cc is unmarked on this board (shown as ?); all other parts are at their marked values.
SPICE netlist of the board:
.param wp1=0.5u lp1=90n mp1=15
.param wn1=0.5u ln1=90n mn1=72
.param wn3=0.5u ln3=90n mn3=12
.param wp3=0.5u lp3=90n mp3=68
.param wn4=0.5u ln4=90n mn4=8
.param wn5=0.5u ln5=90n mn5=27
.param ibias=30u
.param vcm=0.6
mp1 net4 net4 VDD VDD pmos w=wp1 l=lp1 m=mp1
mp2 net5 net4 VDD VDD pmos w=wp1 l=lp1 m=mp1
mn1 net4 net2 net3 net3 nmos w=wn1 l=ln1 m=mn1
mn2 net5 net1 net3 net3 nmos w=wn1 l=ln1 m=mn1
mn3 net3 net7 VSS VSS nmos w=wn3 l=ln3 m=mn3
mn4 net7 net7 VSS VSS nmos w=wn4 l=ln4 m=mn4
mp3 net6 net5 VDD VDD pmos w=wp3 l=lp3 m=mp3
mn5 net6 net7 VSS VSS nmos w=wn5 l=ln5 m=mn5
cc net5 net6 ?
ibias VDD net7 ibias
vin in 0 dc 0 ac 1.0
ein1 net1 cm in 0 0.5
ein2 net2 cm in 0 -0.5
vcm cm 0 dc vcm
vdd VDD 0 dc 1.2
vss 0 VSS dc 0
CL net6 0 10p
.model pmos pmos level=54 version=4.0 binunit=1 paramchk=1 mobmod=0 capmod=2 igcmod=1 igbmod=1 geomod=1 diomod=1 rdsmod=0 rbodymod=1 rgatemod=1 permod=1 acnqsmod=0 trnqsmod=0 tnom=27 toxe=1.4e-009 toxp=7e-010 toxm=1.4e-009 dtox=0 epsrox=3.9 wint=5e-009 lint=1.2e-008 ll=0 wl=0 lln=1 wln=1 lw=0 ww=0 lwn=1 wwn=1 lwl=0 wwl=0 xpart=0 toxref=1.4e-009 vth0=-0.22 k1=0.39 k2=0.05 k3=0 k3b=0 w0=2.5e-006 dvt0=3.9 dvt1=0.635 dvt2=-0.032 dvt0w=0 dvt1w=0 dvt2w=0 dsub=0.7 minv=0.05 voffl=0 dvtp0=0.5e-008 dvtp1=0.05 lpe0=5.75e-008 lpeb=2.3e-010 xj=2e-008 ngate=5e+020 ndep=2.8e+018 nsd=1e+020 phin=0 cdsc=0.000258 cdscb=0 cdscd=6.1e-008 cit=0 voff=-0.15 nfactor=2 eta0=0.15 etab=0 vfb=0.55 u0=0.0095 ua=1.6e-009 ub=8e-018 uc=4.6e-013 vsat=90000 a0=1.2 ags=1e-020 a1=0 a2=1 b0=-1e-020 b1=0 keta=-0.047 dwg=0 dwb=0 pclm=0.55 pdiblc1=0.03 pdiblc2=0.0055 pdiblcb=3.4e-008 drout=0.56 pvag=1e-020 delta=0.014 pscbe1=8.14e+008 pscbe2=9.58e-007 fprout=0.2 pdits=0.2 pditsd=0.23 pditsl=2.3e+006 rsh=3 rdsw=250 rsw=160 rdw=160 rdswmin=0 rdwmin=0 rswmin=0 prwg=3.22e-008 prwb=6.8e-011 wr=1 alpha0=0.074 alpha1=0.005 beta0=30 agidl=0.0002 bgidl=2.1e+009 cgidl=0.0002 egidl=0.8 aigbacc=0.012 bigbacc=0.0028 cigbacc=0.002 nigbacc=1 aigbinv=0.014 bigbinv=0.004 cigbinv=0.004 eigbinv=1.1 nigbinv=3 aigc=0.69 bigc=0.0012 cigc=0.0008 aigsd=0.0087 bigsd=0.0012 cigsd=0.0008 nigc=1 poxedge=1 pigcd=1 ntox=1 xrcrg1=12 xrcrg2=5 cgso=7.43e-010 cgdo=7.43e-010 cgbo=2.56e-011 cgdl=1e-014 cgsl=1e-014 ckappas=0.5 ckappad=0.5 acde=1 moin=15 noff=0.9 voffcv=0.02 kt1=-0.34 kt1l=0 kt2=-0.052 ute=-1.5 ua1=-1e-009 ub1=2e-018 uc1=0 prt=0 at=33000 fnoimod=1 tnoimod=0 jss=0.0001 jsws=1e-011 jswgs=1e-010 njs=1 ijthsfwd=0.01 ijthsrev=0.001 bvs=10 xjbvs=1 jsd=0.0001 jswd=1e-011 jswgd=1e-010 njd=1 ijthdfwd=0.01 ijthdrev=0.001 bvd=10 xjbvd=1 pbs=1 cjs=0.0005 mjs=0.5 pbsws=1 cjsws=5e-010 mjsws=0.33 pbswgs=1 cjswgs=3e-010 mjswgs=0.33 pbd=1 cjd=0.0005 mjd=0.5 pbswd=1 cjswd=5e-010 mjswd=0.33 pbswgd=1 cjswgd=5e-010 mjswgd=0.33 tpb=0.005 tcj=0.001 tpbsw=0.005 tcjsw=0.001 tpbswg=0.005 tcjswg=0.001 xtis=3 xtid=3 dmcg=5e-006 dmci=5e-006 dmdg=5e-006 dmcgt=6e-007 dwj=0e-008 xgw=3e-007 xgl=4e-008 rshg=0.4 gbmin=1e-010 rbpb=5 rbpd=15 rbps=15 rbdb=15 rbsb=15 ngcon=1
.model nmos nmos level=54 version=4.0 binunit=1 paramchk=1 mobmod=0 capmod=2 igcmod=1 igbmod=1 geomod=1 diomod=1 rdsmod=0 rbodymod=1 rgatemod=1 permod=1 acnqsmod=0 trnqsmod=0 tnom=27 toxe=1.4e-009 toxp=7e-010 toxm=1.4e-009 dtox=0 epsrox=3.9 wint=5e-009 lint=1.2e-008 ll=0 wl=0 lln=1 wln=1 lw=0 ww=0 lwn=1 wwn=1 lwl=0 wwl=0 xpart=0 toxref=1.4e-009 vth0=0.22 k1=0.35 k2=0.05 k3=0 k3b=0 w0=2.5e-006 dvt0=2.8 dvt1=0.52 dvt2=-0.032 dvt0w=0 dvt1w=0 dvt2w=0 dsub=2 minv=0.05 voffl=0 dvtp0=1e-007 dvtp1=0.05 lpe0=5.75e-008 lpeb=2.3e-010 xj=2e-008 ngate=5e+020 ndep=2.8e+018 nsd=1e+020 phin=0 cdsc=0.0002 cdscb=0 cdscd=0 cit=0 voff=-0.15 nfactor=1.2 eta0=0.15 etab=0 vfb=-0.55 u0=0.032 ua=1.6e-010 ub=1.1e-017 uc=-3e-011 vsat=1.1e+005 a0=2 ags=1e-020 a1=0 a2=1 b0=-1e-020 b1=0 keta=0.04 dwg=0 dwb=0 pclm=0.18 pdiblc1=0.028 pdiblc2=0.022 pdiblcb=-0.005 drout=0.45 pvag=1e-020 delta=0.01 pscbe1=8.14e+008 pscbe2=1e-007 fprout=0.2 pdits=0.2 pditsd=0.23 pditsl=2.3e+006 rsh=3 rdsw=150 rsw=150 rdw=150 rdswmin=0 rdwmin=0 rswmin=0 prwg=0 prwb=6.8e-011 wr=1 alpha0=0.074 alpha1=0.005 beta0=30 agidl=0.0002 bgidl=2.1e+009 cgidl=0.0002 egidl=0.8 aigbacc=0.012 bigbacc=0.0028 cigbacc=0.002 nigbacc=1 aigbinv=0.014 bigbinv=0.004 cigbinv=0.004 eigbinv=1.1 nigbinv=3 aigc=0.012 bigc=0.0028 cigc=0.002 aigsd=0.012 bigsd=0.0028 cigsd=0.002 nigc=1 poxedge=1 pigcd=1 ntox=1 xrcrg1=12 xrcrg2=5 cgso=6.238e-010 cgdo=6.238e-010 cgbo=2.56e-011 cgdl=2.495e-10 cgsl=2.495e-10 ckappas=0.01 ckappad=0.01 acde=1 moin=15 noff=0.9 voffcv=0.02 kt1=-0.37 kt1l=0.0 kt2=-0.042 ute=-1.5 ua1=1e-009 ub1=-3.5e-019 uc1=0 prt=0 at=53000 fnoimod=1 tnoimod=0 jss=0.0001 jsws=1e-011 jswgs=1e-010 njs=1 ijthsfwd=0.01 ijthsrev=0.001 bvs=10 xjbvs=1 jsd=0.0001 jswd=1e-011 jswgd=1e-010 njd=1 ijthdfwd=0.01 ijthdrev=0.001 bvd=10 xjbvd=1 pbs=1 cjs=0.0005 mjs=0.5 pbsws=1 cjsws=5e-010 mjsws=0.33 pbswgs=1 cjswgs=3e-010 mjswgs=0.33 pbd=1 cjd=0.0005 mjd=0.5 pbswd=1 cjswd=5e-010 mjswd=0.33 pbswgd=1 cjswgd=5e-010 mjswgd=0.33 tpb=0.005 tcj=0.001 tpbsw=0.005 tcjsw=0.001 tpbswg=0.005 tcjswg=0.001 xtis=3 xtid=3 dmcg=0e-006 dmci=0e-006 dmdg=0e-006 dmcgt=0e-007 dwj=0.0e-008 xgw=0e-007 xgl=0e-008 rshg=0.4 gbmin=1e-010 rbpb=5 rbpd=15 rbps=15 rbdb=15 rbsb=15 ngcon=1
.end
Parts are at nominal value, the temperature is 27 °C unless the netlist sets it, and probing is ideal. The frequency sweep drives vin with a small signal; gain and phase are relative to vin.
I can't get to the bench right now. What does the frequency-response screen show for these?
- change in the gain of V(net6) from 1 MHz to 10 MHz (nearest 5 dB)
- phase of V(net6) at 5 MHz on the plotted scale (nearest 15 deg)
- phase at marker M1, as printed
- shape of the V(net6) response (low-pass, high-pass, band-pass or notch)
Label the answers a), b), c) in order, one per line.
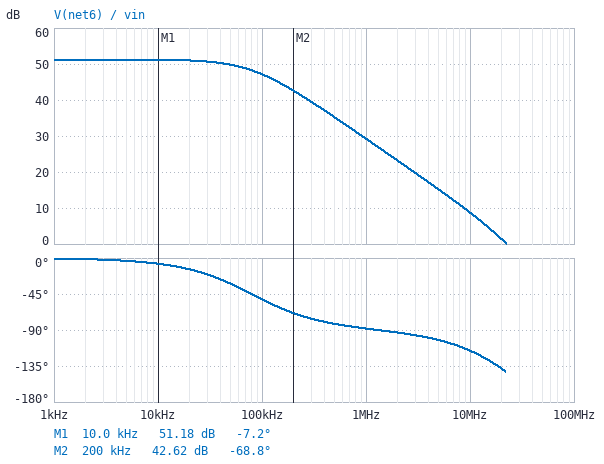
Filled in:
a) -20 dB
b) -105 deg
c) -7.2 deg
d) low-pass
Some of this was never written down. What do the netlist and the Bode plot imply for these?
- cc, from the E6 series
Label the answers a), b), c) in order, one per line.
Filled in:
a) 2.2 pF
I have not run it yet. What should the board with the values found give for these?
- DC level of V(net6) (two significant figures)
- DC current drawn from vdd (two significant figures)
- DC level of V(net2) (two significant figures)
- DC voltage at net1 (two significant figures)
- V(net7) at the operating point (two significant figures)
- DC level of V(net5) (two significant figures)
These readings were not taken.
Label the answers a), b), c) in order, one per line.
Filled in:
a) 520 mV
b) 180 µA
c) 600 mV
d) 600 mV
e) 390 mV
f) 820 mV
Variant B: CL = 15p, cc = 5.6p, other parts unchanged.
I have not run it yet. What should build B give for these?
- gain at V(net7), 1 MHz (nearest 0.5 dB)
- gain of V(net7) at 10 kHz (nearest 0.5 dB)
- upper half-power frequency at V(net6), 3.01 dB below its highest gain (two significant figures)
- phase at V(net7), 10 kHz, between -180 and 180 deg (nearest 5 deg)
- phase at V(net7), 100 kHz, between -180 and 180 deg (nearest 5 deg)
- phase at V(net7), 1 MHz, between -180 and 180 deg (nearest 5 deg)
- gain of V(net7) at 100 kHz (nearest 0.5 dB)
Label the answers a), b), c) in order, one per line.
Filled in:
a) -51.5 dB
b) -24.5 dB
c) 32 kHz
d) -15 deg
e) -70 deg
f) -55 deg
g) -34.0 dB
